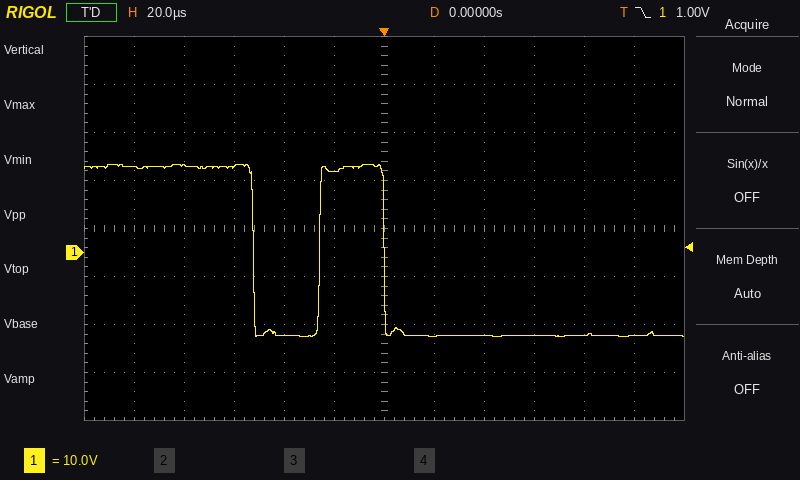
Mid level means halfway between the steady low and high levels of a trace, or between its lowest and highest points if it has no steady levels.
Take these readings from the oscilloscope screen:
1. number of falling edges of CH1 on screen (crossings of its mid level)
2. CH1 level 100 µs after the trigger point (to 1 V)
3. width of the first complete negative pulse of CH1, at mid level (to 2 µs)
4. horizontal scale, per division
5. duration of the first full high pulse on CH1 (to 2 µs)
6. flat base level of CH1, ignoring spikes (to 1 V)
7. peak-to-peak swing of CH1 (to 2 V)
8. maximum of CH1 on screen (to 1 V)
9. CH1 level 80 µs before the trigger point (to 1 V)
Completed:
2
-17 V
26 µs
20 µs
26 µs
-17 V
36 V
18 V
18 V
